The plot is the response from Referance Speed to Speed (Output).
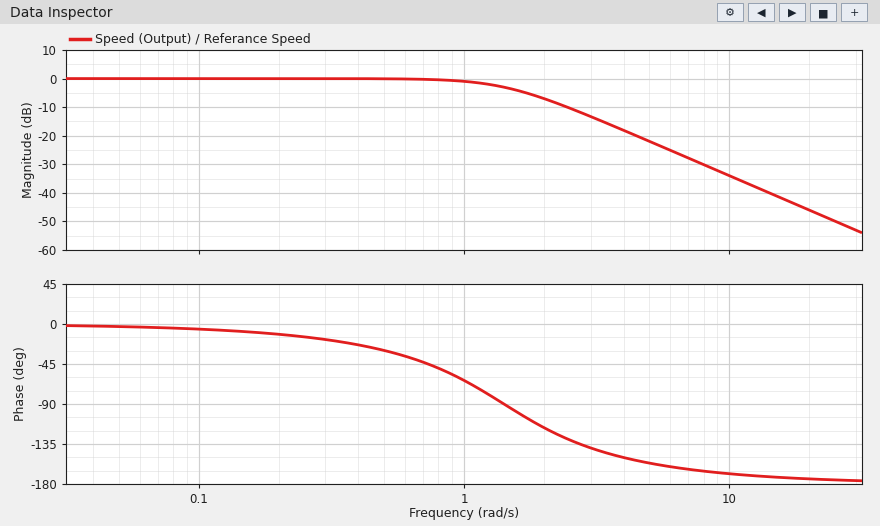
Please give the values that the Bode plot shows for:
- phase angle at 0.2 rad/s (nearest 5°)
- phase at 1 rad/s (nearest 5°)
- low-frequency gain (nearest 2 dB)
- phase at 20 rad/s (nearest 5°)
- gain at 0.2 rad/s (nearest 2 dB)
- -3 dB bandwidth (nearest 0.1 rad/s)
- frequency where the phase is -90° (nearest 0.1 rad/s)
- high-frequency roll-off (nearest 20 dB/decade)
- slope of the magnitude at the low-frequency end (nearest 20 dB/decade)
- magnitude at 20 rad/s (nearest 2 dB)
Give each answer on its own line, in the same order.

-10°
-65°
0 dB
-175°
0 dB
1.4 rad/s
1.4 rad/s
-40 dB/decade
0 dB/decade
-46 dB
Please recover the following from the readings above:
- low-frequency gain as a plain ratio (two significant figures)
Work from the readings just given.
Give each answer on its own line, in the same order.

1.0
